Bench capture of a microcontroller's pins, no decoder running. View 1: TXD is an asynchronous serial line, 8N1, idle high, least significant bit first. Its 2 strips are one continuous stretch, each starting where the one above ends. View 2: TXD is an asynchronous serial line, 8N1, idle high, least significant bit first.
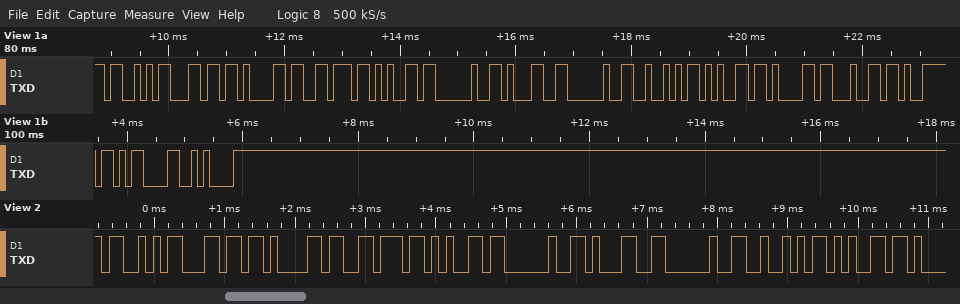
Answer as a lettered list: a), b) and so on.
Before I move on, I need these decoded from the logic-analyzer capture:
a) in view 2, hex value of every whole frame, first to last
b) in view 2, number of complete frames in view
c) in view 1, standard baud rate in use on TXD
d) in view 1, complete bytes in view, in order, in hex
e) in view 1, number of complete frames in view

a) 53 6C 61 76 65 20 31 20 52 65
b) 10
c) 9600 baud
d) 53 6C 61 76 65 20 31 20 52 65 61 64 79 0D 0A
e) 15
